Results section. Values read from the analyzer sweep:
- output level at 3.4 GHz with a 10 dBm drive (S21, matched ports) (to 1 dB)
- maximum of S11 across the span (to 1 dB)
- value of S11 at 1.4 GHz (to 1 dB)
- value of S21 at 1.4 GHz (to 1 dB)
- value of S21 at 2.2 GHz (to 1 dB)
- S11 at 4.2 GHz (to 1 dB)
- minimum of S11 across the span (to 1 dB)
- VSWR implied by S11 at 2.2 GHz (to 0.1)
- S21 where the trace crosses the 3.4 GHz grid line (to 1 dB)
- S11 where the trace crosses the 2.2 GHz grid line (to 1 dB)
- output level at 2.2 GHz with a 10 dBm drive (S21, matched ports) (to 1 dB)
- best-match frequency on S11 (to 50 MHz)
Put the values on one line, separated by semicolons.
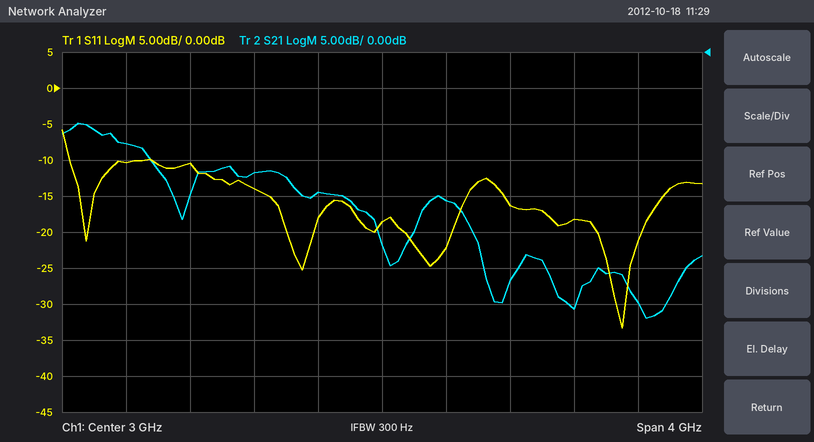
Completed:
-11 dBm; -6 dB; -10 dB; -13 dB; -17 dB; -18 dB; -33 dB; 1.5; -21 dB; -14 dB; -7 dBm; 4.50 GHz
